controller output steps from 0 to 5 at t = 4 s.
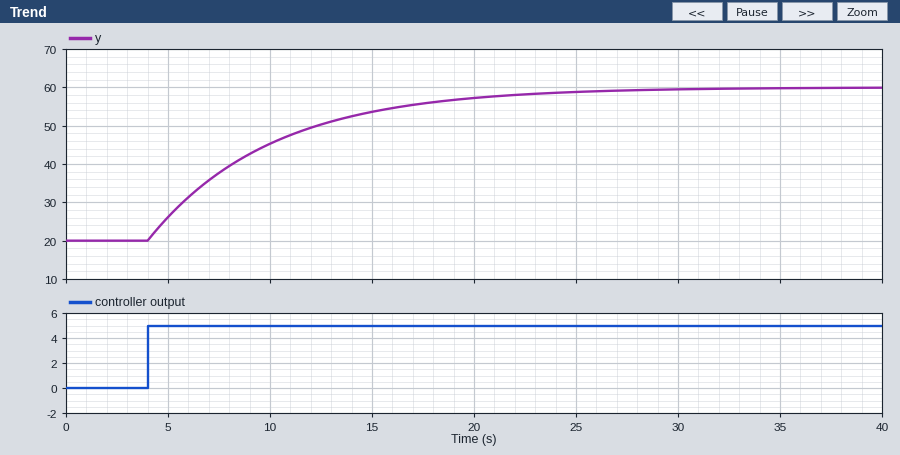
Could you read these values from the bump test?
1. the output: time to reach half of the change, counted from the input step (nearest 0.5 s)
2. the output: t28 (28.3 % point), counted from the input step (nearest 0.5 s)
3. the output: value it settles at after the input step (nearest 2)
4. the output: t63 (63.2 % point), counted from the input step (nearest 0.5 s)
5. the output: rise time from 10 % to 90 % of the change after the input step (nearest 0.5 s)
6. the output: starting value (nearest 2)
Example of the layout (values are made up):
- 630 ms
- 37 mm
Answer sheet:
- 4.0 s
- 2.0 s
- 60
- 6.0 s
- 13.0 s
- 20
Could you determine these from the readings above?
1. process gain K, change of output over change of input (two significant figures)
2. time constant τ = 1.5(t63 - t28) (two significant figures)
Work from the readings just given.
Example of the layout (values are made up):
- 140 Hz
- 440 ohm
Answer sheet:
- 8.0
- 6.0 s
